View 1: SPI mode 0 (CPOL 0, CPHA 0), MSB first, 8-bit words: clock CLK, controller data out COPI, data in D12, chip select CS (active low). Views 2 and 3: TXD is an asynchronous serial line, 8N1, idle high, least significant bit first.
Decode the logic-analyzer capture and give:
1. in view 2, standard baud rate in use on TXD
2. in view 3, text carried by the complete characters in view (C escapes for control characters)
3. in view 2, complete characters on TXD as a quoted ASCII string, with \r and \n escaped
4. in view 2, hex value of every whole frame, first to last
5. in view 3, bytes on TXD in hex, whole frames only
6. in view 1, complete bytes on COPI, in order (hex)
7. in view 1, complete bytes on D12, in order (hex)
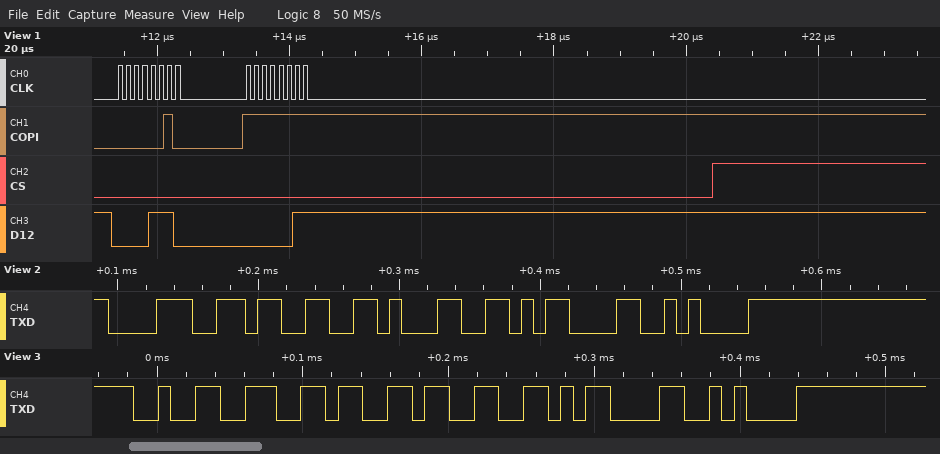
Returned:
115200 baud
"263\r\n"
"831\r\n"
0x38 0x33 0x31 0x0D 0x0A
0x32 0x36 0x33 0x0D 0x0A
02 FF
0E 03
